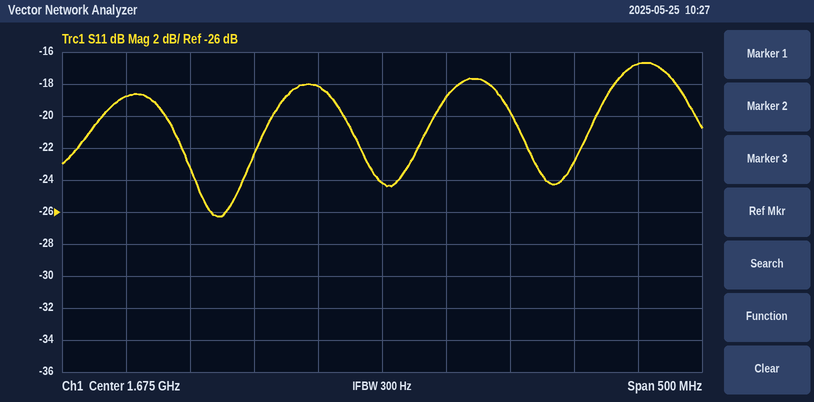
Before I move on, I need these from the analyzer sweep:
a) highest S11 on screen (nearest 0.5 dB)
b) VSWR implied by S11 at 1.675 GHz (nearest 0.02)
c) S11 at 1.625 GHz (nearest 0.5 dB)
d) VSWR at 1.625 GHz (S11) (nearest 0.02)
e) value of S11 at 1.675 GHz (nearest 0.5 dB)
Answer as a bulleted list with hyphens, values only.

- -16.5 dB
- 1.14
- -18.0 dB
- 1.28
- -24.0 dB
